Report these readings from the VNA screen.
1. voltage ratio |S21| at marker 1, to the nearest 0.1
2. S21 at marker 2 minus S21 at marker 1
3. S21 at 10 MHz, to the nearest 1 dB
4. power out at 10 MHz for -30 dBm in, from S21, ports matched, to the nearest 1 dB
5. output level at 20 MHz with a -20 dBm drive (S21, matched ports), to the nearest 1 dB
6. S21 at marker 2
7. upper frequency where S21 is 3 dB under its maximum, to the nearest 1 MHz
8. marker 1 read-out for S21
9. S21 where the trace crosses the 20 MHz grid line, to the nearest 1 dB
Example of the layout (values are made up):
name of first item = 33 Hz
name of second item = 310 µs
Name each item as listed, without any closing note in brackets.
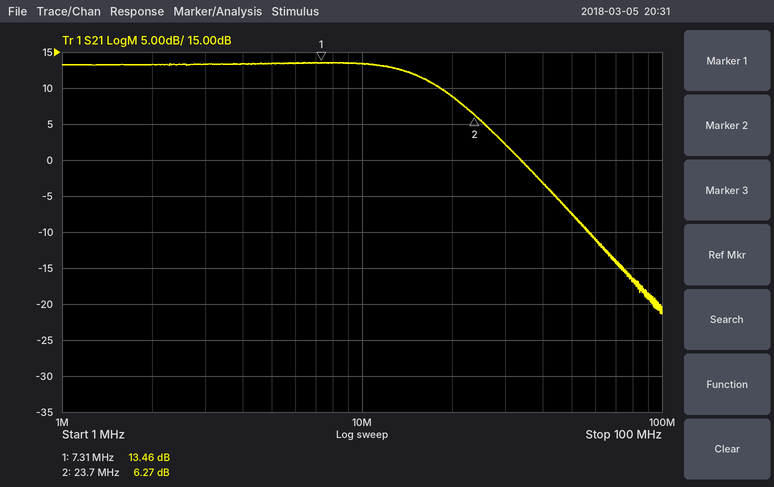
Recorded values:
voltage ratio |S21| at marker 1, to the nearest 0.1 = 4.7
S21 at marker 2 minus S21 at marker 1 = -7.19 dB
S21 at 10 MHz, to the nearest 1 dB = 13 dB
power out at 10 MHz for -30 dBm in, from S21, ports matched, to the nearest 1 dB = -17 dBm
output level at 20 MHz with a -20 dBm drive (S21, matched ports), to the nearest 1 dB = -11 dBm
S21 at marker 2 = 6.27 dB
upper frequency where S21 is 3 dB under its maximum, to the nearest 1 MHz = 17 MHz
marker 1 read-out for S21 = 13.46 dB
S21 where the trace crosses the 20 MHz grid line, to the nearest 1 dB = 9 dB
